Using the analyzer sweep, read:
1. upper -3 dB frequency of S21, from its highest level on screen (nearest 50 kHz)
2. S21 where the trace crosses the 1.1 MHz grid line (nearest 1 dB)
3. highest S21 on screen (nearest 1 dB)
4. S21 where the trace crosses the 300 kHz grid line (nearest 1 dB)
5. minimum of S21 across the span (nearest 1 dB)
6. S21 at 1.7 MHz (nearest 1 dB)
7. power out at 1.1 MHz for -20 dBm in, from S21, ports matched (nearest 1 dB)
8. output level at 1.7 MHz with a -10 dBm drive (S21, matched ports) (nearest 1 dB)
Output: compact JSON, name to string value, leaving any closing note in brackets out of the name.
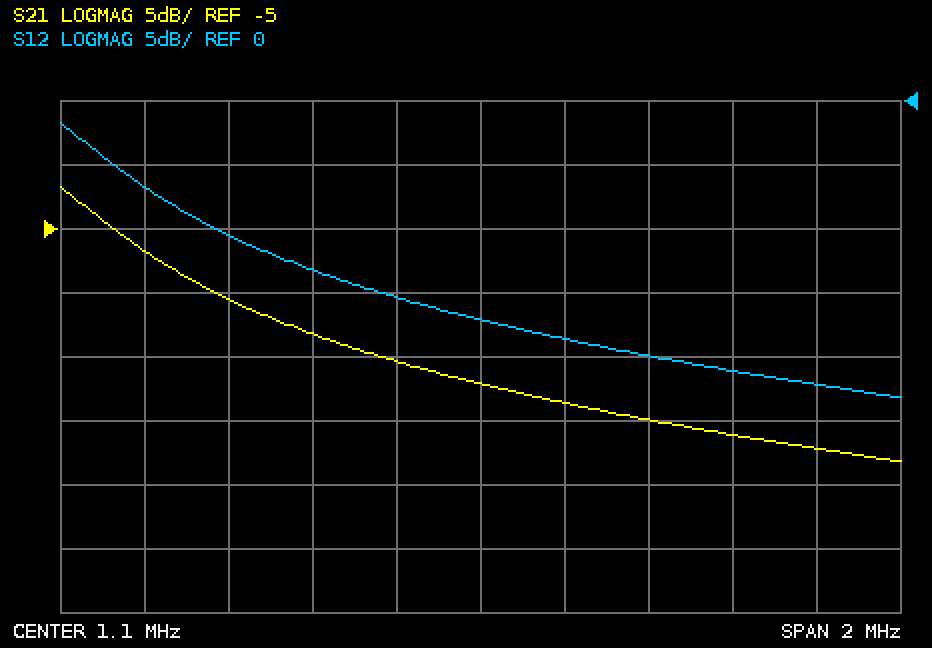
{"upper -3 dB frequency of S21, from its highest level on screen": "200 kHz", "S21 where the trace crosses the 1.1 MHz grid line": "-17 dB", "highest S21 on screen": "-2 dB", "S21 where the trace crosses the 300 kHz grid line": "-7 dB", "minimum of S21 across the span": "-23 dB", "S21 at 1.7 MHz": "-21 dB", "power out at 1.1 MHz for -20 dBm in, from S21, ports matched": "-37 dBm", "output level at 1.7 MHz with a -10 dBm drive (S21, matched ports)": "-31 dBm"}
